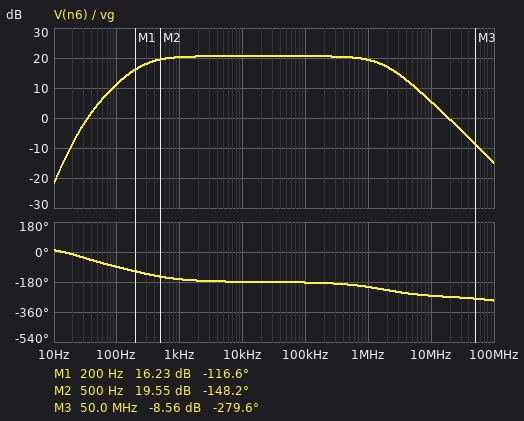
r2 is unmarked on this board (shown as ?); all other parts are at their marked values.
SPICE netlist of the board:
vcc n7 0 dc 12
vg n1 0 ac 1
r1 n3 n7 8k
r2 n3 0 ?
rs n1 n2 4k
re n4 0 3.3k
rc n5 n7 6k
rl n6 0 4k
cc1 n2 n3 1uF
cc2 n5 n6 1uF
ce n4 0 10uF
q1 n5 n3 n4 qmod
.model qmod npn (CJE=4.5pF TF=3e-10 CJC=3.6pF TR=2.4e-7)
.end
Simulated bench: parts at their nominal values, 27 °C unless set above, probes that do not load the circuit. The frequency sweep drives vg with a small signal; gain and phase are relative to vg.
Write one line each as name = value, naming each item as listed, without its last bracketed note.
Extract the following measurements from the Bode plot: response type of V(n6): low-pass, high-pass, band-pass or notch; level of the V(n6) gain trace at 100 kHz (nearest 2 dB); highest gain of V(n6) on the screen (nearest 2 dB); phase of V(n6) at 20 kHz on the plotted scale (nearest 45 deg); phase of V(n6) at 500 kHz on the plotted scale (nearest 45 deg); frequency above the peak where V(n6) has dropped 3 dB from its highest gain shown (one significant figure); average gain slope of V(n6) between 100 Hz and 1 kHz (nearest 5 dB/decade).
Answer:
response type of V(n6): low-pass, high-pass, band-pass or notch = band-pass
level of the V(n6) gain trace at 100 kHz = 20 dB
highest gain of V(n6) on the screen = 20 dB
phase of V(n6) at 20 kHz on the plotted scale = -180 deg
phase of V(n6) at 500 kHz on the plotted scale = -180 deg
frequency above the peak where V(n6) has dropped 3 dB from its highest gain shown = 2 MHz
average gain slope of V(n6) between 100 Hz and 1 kHz = 10 dB/decade
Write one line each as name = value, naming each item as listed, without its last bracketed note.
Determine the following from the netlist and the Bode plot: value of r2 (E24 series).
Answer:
value of r2 = 2 kΩ
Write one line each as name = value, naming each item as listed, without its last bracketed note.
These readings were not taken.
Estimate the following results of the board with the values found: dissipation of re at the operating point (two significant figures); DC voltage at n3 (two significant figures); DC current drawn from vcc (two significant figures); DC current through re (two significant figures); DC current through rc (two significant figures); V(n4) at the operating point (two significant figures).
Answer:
dissipation of re at the operating point = 810 µW
DC voltage at n3 = 2.4 V
DC current drawn from vcc = 1.7 mA
DC current through re = 500 µA
DC current through rc = 490 µA
V(n4) at the operating point = 1.6 V
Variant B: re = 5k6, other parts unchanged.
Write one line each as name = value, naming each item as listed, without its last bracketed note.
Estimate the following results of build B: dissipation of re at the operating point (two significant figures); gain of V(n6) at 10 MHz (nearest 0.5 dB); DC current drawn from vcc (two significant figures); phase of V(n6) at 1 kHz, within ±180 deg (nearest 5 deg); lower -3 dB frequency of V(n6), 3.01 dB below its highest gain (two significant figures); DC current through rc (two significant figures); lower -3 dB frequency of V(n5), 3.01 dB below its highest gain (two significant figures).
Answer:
dissipation of re at the operating point = 490 µW
gain of V(n6) at 10 MHz = 5.0 dB
DC current drawn from vcc = 1.5 mA
phase of V(n6) at 1 kHz, within ±180 deg = -170 deg
lower -3 dB frequency of V(n6), 3.01 dB below its highest gain = 170 Hz
DC current through rc = 290 µA
lower -3 dB frequency of V(n5), 3.01 dB below its highest gain = 160 Hz
